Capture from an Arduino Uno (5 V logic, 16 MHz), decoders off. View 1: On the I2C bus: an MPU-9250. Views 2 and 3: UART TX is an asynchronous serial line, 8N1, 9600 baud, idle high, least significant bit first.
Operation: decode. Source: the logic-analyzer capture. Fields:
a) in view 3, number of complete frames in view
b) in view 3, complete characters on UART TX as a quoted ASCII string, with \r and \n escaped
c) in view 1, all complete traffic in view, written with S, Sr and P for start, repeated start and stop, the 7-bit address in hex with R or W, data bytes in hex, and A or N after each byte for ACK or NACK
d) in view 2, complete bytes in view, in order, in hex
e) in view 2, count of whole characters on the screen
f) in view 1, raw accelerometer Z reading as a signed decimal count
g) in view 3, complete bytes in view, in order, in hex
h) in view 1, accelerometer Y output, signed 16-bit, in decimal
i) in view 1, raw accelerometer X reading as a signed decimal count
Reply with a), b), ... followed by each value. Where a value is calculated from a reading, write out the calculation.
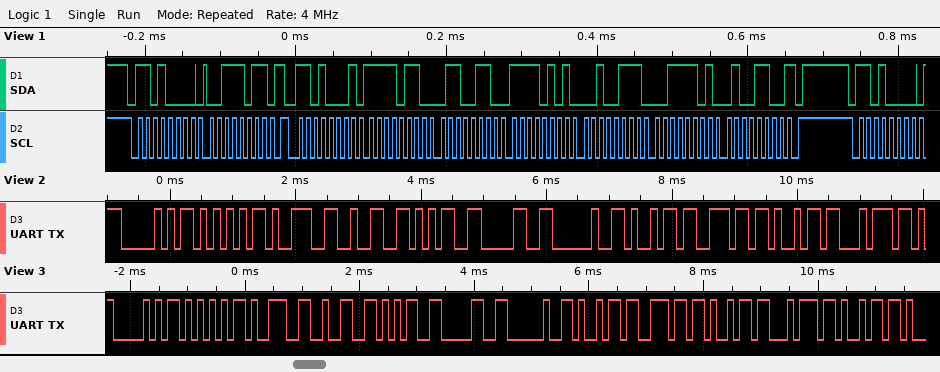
a) 12
b) "PU9250 initi"
c) S 68W A 3B A Sr 68R A F6 A 66 A F5 A 27 A 3D A 4C N P S 68W A
d) 50 55 39 32 35 30 20 69 6E 69 74
e) 11
f) 0x3D4C = 15692
g) 50 55 39 32 35 30 20 69 6E 69 74 69
h) 0xF527 = -2777
i) 0xF666 = -2458
